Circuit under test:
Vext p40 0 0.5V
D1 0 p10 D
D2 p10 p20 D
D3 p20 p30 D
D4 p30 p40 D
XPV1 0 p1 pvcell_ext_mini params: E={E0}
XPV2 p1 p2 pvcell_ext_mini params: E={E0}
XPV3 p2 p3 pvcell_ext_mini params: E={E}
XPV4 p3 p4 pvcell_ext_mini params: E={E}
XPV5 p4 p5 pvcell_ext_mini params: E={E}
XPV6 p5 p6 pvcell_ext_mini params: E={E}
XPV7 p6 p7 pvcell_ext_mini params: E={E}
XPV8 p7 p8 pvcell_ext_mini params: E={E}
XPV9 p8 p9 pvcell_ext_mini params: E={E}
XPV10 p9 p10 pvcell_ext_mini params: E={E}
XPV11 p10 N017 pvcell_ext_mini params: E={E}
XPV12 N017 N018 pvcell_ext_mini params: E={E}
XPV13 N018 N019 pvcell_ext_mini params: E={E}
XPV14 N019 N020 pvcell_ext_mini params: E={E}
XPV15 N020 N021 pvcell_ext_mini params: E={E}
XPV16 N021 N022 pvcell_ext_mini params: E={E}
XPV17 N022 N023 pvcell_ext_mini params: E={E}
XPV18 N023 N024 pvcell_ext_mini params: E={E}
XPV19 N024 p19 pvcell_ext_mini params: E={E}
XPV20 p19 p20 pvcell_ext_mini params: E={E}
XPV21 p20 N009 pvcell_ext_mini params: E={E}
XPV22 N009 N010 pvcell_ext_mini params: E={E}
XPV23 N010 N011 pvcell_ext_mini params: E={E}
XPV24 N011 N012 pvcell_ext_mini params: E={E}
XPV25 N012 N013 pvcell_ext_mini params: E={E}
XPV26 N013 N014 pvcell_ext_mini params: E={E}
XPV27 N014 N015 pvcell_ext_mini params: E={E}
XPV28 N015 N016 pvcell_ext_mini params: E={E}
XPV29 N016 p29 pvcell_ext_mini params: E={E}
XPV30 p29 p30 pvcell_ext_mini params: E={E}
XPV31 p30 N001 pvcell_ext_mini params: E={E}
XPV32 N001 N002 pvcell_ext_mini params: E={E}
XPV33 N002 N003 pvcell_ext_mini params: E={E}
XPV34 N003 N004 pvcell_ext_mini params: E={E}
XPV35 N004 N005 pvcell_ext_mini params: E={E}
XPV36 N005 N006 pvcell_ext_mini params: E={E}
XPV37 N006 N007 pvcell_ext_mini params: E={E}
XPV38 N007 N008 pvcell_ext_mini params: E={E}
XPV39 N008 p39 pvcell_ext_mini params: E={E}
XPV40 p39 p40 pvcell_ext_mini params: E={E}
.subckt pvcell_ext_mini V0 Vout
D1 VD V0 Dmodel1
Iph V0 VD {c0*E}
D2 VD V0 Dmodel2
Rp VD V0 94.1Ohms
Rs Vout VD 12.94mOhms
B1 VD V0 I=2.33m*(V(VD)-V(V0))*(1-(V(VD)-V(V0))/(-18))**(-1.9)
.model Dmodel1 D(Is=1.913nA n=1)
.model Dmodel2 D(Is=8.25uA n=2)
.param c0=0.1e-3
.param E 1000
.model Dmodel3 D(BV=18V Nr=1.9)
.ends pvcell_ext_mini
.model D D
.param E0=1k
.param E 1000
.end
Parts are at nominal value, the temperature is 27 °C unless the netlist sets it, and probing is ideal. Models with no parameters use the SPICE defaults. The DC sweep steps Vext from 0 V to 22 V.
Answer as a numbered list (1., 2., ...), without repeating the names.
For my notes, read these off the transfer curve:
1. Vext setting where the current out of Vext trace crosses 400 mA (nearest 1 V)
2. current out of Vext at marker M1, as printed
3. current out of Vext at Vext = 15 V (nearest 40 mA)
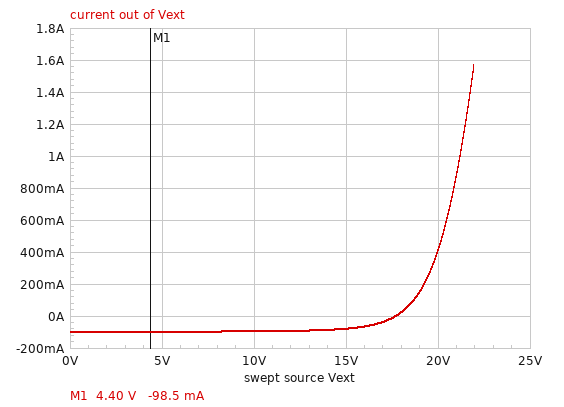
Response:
1. 20 V
2. -98.5 mA
3. -80 mA
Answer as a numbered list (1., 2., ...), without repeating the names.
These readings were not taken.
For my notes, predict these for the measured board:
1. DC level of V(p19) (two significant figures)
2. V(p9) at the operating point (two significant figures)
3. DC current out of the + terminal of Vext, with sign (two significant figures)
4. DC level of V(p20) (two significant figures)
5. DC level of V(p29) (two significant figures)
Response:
1. 240 mV
2. 110 mV
3. -100 mA
4. 250 mV
5. 360 mV
